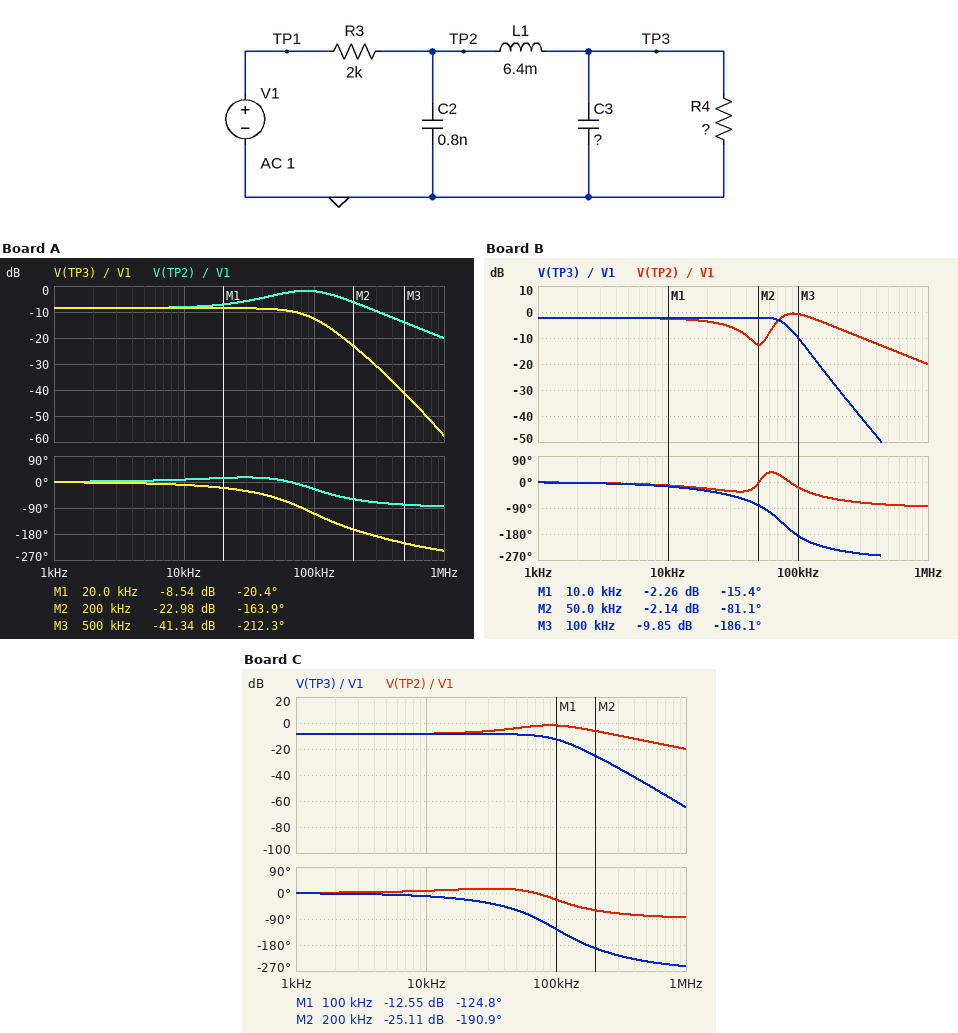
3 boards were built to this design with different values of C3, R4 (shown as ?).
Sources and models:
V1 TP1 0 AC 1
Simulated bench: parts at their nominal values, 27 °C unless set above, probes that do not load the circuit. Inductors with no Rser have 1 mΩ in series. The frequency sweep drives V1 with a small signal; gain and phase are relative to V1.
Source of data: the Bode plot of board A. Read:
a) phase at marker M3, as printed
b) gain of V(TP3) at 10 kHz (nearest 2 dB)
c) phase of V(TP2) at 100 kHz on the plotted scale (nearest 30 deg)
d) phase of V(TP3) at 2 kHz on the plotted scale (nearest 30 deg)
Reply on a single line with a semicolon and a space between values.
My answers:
-212.3 deg; -8 dB; -30 deg; 0 deg
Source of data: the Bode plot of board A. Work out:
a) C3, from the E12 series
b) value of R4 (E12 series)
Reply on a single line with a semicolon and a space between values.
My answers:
270 pF; 1.2 kΩ
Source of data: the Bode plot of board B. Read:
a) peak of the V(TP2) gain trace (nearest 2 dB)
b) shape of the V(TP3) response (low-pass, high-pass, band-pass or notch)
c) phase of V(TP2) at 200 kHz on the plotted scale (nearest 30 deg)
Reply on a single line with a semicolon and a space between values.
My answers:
0 dB; low-pass; -60 deg
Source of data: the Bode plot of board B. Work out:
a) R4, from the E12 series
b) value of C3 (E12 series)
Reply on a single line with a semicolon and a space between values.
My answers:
6.8 kΩ; 1.5 nF
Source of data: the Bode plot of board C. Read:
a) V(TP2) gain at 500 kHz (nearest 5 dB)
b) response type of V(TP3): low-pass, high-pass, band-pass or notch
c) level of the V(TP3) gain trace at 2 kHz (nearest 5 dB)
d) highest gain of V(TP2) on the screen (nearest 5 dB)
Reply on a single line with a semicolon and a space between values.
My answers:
-15 dB; low-pass; -10 dB; 0 dB
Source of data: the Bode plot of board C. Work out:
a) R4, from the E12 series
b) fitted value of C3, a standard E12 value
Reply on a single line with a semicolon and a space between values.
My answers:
1.2 kΩ; 680 pF
